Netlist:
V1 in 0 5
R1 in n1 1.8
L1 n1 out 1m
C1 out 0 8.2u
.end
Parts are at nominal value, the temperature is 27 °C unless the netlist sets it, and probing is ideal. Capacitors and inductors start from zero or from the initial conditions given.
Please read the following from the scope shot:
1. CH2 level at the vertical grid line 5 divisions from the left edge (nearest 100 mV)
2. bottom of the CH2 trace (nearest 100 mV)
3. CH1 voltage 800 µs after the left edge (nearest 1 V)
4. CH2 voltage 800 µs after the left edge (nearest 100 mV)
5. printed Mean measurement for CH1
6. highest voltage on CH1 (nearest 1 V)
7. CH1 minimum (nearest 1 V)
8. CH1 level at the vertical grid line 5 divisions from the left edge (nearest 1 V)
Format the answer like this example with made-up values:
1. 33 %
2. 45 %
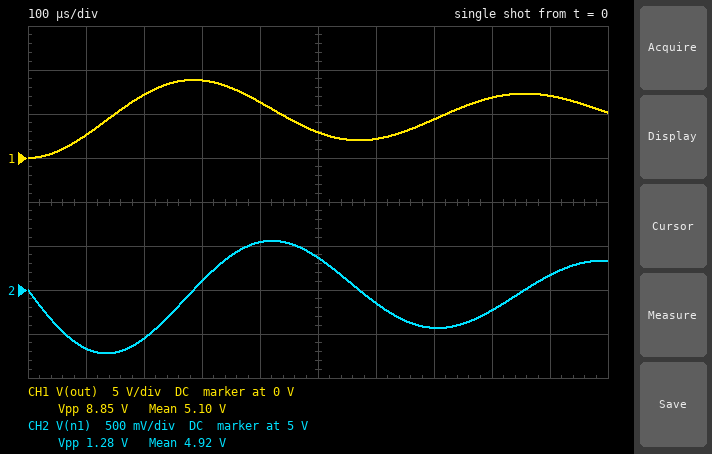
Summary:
1. 5.4 V
2. 4.3 V
3. 7 V
4. 4.8 V
5. 5.10 V
6. 9 V
7. 0 V
8. 3 V
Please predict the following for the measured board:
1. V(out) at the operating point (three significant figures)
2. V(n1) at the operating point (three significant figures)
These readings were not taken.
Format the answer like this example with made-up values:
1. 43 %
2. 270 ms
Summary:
1. 5.00 V
2. 5.00 V
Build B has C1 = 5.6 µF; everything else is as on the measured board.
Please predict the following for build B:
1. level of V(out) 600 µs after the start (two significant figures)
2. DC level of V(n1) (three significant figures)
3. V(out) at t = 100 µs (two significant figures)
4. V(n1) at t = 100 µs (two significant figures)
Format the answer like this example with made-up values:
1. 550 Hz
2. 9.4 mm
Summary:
1. 5.2 V
2. 5.00 V
3. 3.6 V
4. 4.4 V
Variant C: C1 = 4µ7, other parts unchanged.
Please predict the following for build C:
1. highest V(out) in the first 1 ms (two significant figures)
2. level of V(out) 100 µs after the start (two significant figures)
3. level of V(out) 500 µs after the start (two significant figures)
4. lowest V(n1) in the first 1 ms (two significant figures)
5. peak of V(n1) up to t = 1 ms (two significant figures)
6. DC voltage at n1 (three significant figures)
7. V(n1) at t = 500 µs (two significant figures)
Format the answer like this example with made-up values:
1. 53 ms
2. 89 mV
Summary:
1. 9.1 V
2. 4.2 V
3. 3.1 V
4. 4.4 V
5. 5.5 V
6. 5.00 V
7. 4.7 V
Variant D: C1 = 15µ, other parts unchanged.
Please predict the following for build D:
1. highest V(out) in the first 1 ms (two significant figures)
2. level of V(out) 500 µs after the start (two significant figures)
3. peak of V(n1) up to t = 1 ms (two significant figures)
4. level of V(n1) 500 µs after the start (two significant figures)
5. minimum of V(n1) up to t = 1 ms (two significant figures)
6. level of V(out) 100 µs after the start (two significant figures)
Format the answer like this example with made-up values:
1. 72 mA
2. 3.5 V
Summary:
1. 8.5 V
2. 7.2 V
3. 5.7 V
4. 5.6 V
5. 4.1 V
6. 1.5 V
